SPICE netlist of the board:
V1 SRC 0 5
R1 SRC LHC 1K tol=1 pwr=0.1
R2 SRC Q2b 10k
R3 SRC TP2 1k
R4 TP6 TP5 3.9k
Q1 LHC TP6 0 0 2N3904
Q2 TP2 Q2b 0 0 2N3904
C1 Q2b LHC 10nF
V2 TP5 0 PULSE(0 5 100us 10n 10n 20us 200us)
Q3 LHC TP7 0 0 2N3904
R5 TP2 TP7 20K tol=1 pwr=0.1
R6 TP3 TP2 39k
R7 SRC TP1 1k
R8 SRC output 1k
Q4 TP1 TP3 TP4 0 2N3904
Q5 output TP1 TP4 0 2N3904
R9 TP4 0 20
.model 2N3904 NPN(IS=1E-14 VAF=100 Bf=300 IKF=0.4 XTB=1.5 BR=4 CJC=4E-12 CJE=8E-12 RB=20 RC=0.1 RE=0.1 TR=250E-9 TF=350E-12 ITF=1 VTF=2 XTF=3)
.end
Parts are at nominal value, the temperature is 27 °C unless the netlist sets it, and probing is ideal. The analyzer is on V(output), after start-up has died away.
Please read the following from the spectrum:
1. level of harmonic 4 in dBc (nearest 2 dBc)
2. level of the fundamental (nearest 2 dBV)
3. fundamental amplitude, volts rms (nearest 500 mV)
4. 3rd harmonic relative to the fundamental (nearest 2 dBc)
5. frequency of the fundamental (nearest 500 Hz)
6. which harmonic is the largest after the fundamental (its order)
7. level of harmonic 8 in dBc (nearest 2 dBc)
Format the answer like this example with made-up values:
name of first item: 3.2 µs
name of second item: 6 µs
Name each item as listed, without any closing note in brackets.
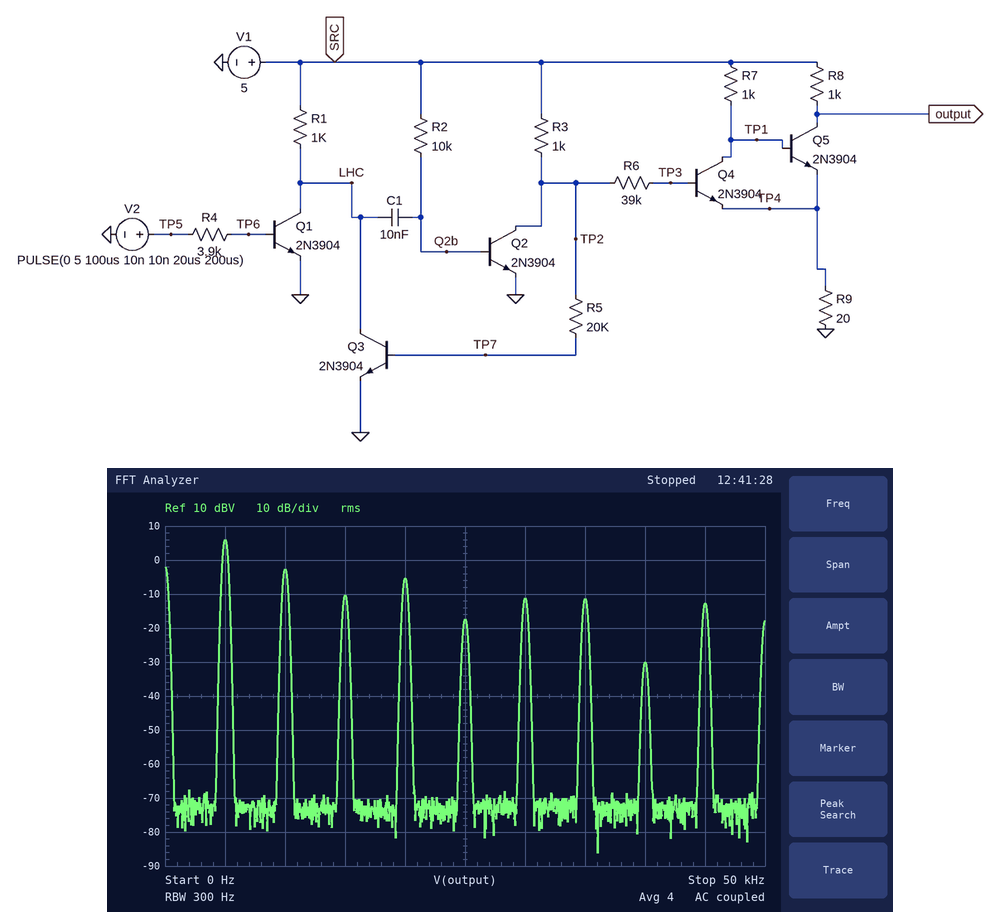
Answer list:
level of harmonic 4 in dBc: -12 dBc
level of the fundamental: 6 dBV
fundamental amplitude, volts rms: 2.0 V
3rd harmonic relative to the fundamental: -16 dBc
frequency of the fundamental: 5.0 kHz
which harmonic is the largest after the fundamental: 2
level of harmonic 8 in dBc: -36 dBc
